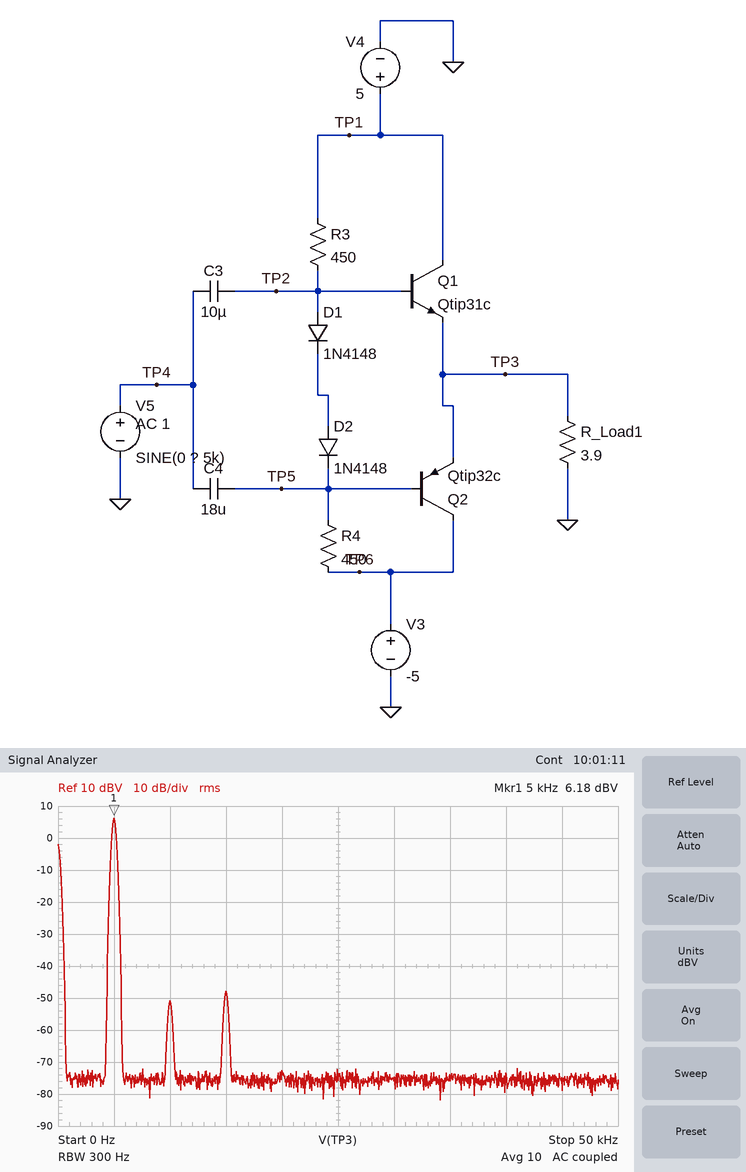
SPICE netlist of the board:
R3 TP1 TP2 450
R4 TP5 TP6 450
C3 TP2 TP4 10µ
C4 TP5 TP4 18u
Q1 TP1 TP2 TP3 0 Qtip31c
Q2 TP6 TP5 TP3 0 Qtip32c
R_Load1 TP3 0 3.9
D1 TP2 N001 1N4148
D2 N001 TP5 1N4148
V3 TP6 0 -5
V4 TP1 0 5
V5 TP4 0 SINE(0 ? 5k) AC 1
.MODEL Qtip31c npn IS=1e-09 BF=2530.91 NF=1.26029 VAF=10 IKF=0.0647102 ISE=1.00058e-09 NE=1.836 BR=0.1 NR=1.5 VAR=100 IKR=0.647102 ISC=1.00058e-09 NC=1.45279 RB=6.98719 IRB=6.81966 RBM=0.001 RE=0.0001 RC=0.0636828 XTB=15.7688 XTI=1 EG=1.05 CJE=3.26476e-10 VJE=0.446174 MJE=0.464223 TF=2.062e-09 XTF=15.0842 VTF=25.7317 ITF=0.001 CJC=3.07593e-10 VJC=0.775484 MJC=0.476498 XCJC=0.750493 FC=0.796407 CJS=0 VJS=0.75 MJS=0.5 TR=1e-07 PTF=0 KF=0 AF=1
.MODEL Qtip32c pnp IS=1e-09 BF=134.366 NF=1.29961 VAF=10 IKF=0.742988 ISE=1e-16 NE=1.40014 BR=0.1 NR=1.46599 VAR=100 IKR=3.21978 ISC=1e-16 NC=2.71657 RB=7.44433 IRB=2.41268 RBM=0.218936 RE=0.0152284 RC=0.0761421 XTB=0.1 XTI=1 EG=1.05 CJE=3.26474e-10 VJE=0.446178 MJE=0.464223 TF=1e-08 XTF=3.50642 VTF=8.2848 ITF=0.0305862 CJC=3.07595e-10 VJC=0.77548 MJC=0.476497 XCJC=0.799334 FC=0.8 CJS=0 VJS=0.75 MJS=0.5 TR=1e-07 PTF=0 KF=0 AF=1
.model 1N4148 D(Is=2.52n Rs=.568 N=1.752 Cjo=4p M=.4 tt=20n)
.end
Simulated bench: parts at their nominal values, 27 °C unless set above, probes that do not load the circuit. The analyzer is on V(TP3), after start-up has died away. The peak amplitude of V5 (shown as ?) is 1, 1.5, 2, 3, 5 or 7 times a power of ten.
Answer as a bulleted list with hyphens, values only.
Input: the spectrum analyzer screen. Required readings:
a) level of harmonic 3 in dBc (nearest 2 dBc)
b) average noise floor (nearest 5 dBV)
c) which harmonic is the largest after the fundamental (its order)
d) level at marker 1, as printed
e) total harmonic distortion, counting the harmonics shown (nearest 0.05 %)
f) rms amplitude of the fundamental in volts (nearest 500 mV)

- -54 dBc
- -75 dBV
- 3
- 6.18 dBV
- 0.25 %
- 2.0 V
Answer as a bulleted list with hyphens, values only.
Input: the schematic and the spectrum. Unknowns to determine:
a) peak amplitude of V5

- 3 V
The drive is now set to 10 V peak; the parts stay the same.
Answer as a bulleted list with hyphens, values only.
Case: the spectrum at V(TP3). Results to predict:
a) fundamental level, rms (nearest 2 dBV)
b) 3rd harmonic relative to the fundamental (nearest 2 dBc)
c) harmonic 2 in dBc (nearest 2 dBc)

- 10 dBV
- -14 dBc
- -42 dBc
